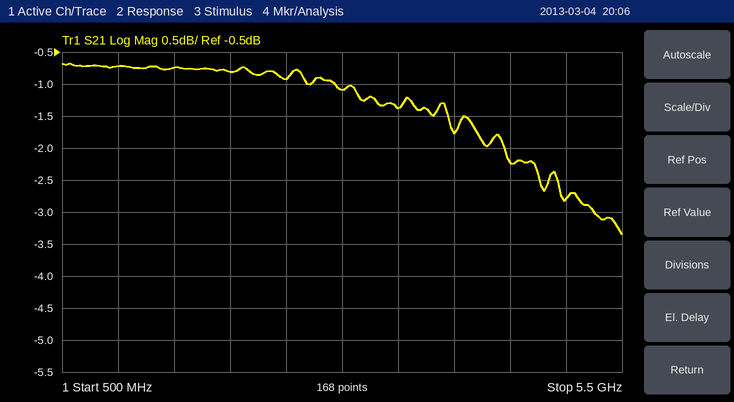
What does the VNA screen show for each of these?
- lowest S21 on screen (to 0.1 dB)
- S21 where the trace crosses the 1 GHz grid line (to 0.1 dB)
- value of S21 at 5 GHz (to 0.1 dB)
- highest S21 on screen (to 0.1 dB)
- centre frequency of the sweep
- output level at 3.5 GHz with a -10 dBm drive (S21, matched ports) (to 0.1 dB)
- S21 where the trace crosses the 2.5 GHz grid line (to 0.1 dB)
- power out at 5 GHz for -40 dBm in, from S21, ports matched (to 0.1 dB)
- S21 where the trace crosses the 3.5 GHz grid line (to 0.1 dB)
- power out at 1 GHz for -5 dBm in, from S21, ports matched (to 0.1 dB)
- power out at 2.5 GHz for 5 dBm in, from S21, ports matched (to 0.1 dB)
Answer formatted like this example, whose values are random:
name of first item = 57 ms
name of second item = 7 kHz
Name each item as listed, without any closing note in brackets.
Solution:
lowest S21 on screen = -3.3 dB
S21 where the trace crosses the 1 GHz grid line = -0.7 dB
value of S21 at 5 GHz = -2.8 dB
highest S21 on screen = -0.7 dB
centre frequency of the sweep = 3 GHz
output level at 3.5 GHz with a -10 dBm drive (S21, matched ports) = -11.4 dBm
S21 where the trace crosses the 2.5 GHz grid line = -0.9 dB
power out at 5 GHz for -40 dBm in, from S21, ports matched = -42.8 dBm
S21 where the trace crosses the 3.5 GHz grid line = -1.4 dB
power out at 1 GHz for -5 dBm in, from S21, ports matched = -5.7 dBm
power out at 2.5 GHz for 5 dBm in, from S21, ports matched = 4.1 dBm
